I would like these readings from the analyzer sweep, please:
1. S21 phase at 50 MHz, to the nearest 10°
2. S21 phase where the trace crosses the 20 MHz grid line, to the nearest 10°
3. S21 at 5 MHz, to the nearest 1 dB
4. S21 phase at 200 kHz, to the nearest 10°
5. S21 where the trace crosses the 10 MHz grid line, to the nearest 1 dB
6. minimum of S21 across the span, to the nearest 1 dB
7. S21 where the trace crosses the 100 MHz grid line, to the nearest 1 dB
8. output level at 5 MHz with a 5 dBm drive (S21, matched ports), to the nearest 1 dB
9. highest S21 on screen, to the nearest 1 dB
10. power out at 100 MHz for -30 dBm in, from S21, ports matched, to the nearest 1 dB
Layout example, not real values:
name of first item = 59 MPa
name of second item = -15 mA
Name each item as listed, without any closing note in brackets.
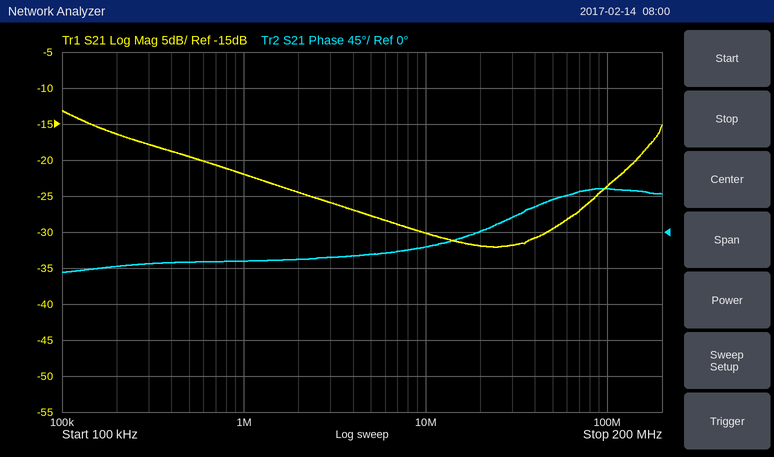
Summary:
S21 phase at 50 MHz, to the nearest 10° = 40°
S21 phase where the trace crosses the 20 MHz grid line, to the nearest 10° = 0°
S21 at 5 MHz, to the nearest 1 dB = -28 dB
S21 phase at 200 kHz, to the nearest 10° = -40°
S21 where the trace crosses the 10 MHz grid line, to the nearest 1 dB = -30 dB
minimum of S21 across the span, to the nearest 1 dB = -32 dB
S21 where the trace crosses the 100 MHz grid line, to the nearest 1 dB = -24 dB
output level at 5 MHz with a 5 dBm drive (S21, matched ports), to the nearest 1 dB = -23 dBm
highest S21 on screen, to the nearest 1 dB = -13 dB
power out at 100 MHz for -30 dBm in, from S21, ports matched, to the nearest 1 dB = -54 dBm
